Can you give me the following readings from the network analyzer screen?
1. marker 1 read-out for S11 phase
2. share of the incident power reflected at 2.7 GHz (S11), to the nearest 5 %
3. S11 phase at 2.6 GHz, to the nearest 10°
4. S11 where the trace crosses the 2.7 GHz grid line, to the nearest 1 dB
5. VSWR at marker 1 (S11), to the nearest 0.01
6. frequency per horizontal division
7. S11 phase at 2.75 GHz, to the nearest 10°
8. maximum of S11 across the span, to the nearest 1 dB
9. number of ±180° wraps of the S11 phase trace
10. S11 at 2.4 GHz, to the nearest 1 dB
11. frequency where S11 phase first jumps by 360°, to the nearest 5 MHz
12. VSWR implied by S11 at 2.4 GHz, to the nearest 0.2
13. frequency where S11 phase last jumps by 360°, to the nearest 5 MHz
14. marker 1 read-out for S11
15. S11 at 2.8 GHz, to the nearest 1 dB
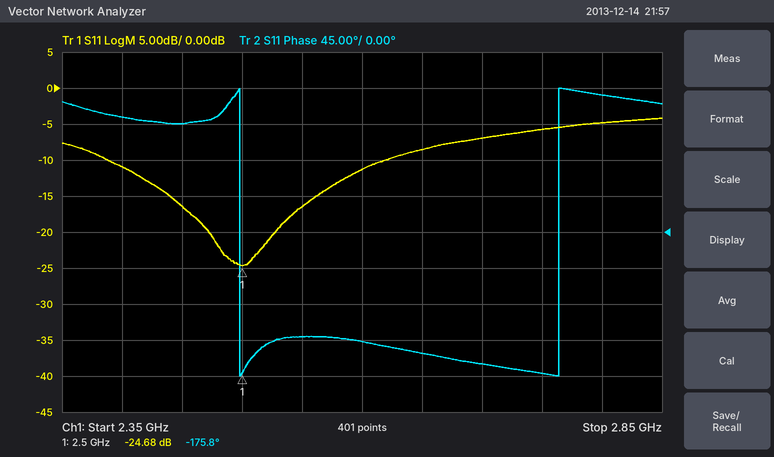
-175.8°
20 %
-140°
-7 dB
1.12
50 MHz
-180°
-4 dB
2
-11 dB
2.500 GHz
1.8
2.765 GHz
-24.68 dB
-5 dB
